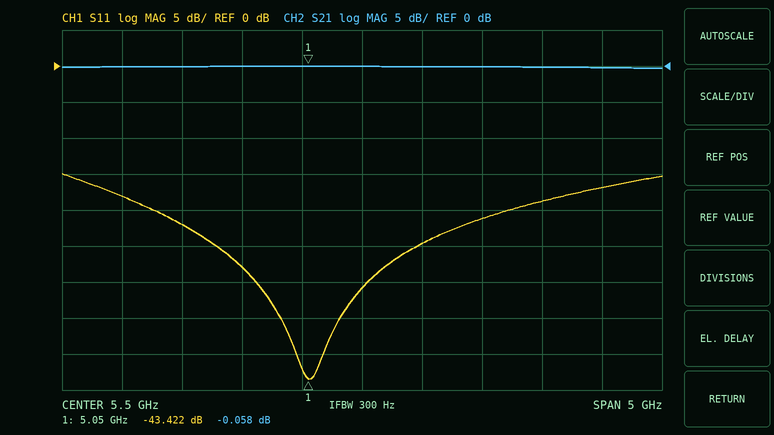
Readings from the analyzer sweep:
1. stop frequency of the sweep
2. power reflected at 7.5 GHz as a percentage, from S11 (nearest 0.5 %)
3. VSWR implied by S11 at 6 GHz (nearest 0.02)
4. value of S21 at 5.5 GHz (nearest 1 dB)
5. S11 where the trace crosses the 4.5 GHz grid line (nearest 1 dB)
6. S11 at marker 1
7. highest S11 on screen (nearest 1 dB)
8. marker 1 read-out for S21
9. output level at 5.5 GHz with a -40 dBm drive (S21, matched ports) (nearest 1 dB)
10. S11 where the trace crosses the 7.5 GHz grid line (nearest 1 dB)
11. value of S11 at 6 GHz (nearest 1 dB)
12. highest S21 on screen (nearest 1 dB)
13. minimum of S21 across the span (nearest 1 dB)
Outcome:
8 GHz
2.0 %
1.12
0 dB
-28 dB
-43.422 dB
-15 dB
-0.058 dB
-40 dBm
-17 dB
-25 dB
0 dB
0 dB
